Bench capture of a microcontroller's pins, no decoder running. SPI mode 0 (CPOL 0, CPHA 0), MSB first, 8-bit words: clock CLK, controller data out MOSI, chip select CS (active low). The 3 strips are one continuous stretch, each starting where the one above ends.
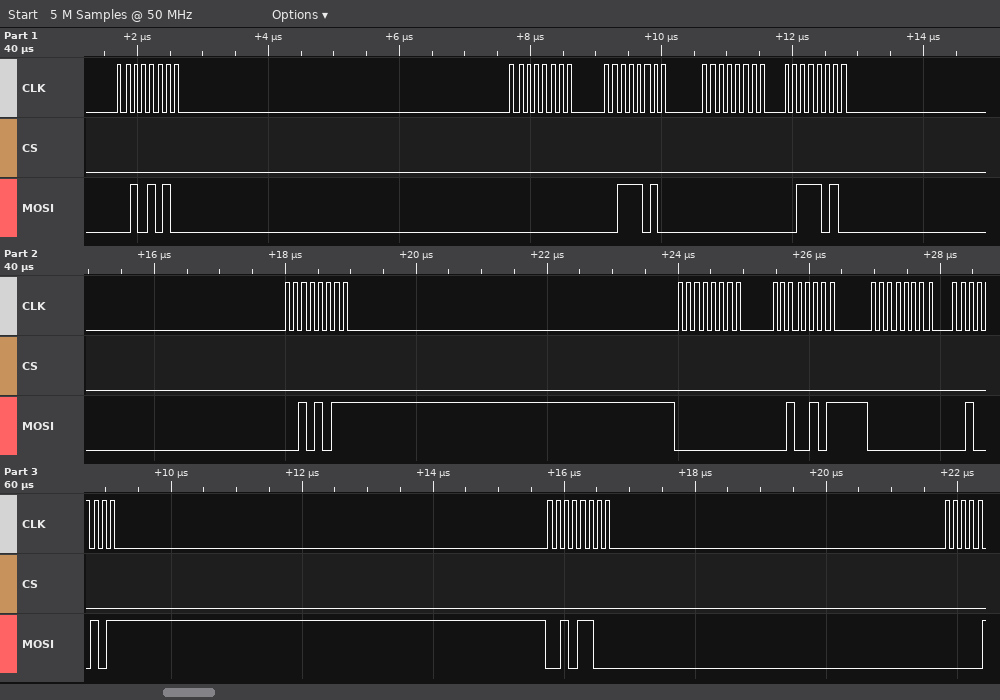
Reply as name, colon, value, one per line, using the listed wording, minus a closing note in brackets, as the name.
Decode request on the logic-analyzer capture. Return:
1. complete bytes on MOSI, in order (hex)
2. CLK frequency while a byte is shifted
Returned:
complete bytes on MOSI, in order: 0x2A 0x00 0x3A 0x00 0x3A 0x2B 0x00 0x25 0x00 0x25 0x2C
CLK frequency while a byte is shifted: 8 MHz
